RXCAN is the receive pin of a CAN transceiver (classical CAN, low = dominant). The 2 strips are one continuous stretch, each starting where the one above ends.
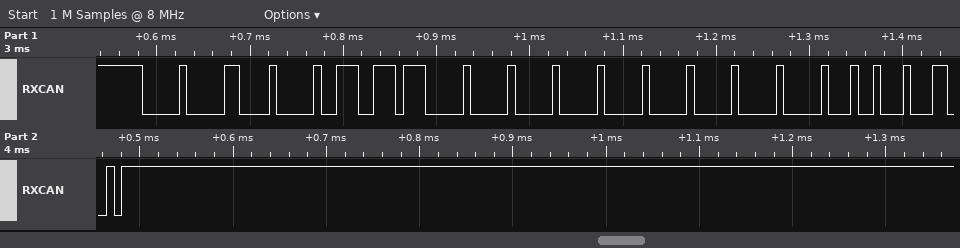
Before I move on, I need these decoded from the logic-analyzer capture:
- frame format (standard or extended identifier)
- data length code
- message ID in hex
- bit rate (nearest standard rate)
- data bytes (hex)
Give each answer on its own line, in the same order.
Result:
standard
8
0x002
125 kbit/s
0E 77 00 00 00 00 00 00
